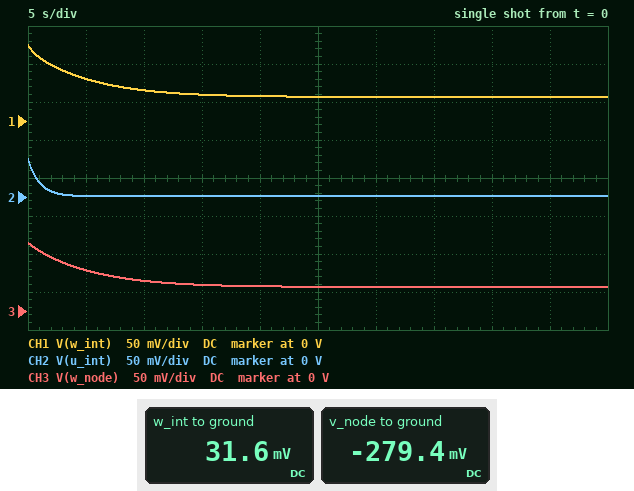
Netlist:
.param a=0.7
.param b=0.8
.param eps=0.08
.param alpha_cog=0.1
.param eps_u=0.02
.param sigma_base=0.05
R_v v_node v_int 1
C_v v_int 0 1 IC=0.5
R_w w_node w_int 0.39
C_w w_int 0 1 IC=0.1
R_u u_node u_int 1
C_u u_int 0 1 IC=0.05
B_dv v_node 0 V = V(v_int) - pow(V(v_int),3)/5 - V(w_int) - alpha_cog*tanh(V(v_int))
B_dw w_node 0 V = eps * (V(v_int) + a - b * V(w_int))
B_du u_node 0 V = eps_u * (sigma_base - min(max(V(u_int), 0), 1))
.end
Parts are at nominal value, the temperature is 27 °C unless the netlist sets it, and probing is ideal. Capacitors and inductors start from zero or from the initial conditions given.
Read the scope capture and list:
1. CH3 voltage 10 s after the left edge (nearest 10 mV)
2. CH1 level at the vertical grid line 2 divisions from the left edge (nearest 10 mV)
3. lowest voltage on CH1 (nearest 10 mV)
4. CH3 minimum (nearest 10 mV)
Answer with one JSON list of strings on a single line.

["40 mV", "40 mV", "30 mV", "30 mV"]
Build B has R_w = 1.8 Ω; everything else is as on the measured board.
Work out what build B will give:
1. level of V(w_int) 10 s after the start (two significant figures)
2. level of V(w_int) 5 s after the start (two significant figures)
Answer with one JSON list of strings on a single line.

["41 mV", "62 mV"]
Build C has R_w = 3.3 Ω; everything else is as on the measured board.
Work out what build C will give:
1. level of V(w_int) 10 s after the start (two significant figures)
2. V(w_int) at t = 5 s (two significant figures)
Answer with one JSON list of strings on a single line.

["45 mV", "69 mV"]
